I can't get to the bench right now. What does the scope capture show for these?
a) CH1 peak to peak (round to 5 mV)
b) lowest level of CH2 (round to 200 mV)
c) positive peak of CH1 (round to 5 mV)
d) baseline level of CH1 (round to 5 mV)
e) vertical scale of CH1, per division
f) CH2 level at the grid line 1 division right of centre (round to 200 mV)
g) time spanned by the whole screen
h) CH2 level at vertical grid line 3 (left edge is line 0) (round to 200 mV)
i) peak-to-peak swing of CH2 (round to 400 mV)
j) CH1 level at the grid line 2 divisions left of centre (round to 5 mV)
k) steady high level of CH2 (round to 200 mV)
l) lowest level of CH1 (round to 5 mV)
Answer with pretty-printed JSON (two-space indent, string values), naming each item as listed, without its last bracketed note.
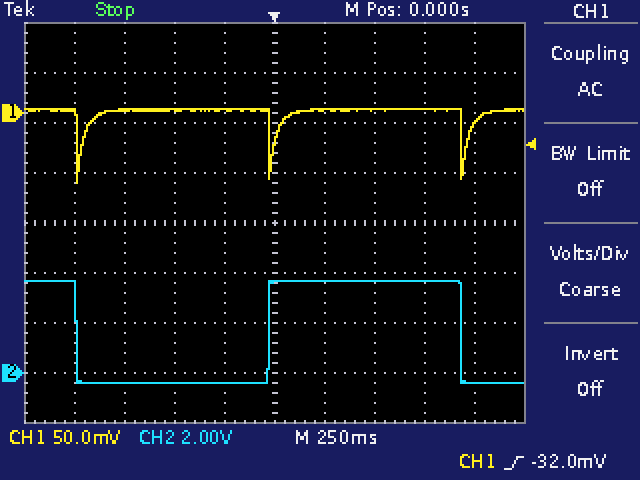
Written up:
{
  "CH1 peak to peak": "75 mV",
  "lowest level of CH2": "-400 mV",
  "positive peak of CH1": "5 mV",
  "baseline level of CH1": "5 mV",
  "vertical scale of CH1, per division": "50 mV",
  "CH2 level at the grid line 1 division right of centre": "3.6 V",
  "time spanned by the whole screen": "2.5 s",
  "CH2 level at vertical grid line 3 (left edge is line 0)": "-400 mV",
  "peak-to-peak swing of CH2": "4.0 V",
  "CH1 level at the grid line 2 divisions left of centre": "5 mV",
  "steady high level of CH2": "3.6 V",
  "lowest level of CH1": "-70 mV"
}
